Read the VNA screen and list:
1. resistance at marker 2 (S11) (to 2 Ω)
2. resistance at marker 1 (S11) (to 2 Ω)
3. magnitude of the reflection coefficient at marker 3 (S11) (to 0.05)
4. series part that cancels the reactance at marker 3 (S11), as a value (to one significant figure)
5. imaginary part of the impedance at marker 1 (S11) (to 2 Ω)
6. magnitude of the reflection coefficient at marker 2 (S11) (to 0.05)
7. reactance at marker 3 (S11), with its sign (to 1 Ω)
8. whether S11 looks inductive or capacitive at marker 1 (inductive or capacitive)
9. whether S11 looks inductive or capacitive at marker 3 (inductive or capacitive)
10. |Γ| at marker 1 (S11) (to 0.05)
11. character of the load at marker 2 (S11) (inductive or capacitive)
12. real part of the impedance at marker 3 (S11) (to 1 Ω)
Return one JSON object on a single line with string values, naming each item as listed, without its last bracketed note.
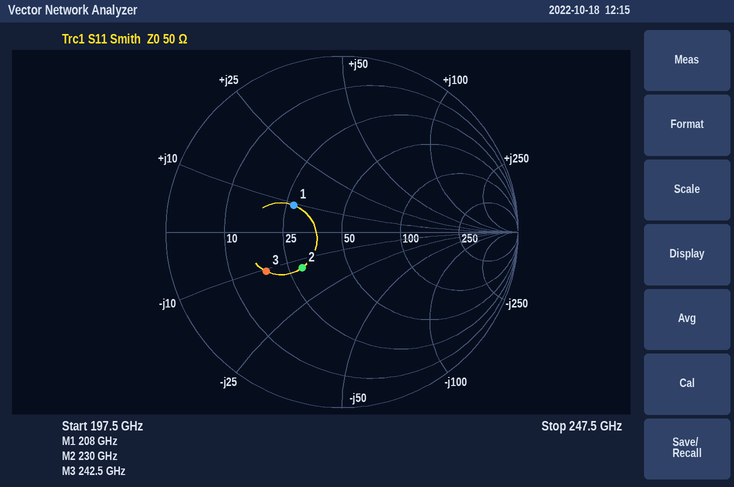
{"resistance at marker 2 (S11)": "30 Ω", "resistance at marker 1 (S11)": "28 Ω", "magnitude of the reflection coefficient at marker 3 (S11)": "0.50", "series part that cancels the reactance at marker 3 (S11), as a value": "7 pH", "imaginary part of the impedance at marker 1 (S11)": "+10 Ω", "magnitude of the reflection coefficient at marker 2 (S11)": "0.30", "reactance at marker 3 (S11), with its sign": "-11 Ω", "whether S11 looks inductive or capacitive at marker 1": "inductive", "whether S11 looks inductive or capacitive at marker 3": "capacitive", "|Γ| at marker 1 (S11)": "0.30", "character of the load at marker 2 (S11)": "capacitive", "real part of the impedance at marker 3 (S11)": "18 Ω"}
